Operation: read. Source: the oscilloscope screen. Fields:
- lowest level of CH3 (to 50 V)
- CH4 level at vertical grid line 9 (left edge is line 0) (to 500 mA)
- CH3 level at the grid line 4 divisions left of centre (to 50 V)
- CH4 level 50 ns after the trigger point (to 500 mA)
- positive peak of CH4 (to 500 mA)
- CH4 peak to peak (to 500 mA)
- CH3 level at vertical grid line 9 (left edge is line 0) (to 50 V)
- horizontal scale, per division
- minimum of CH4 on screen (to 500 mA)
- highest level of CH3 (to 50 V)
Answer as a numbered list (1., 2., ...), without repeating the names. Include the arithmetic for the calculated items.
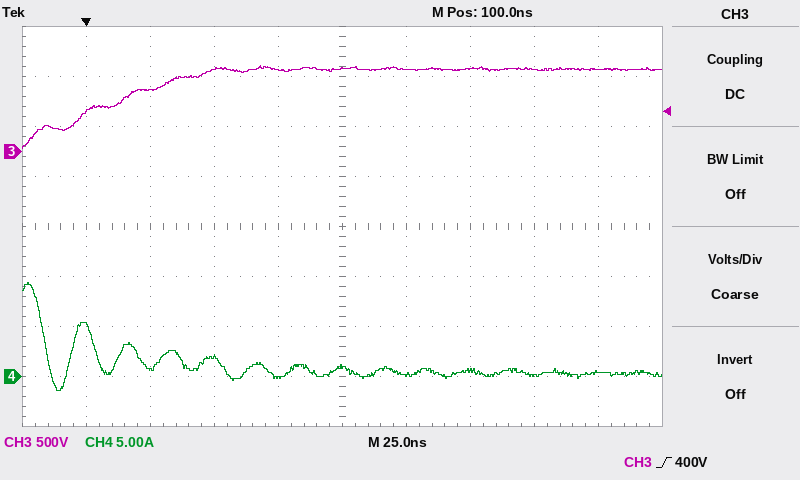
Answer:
1. 50 V
2. 500 mA
3. 400 V
4. 2.0 A
5. 9.5 A
6. 9.5 A − (-1.5 A) = 11.0 A
7. 800 V
8. 25 ns
9. -1.5 A
10. 850 V
